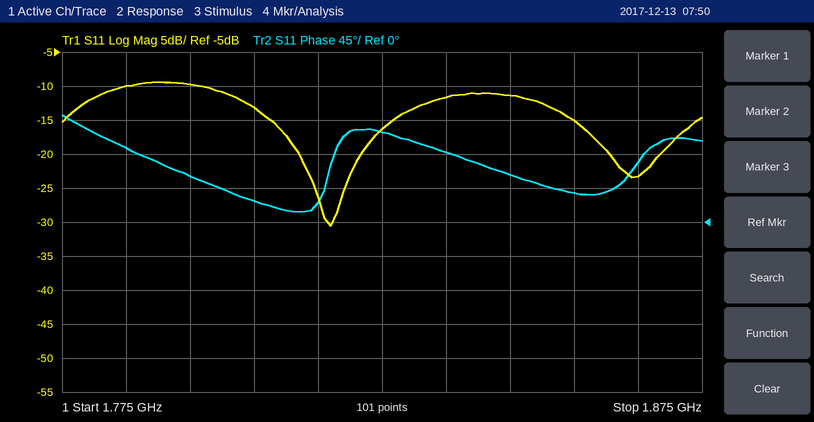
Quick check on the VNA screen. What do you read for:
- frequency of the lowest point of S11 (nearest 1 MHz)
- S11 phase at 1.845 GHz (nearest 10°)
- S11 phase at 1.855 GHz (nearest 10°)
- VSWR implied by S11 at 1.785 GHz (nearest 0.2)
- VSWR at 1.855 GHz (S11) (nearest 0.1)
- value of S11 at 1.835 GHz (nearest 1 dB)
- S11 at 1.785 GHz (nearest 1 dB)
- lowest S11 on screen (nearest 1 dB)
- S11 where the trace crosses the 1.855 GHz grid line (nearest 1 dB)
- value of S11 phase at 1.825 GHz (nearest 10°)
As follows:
1.817 GHz
60°
40°
2.0
1.4
-12 dB
-10 dB
-31 dB
-15 dB
120°
